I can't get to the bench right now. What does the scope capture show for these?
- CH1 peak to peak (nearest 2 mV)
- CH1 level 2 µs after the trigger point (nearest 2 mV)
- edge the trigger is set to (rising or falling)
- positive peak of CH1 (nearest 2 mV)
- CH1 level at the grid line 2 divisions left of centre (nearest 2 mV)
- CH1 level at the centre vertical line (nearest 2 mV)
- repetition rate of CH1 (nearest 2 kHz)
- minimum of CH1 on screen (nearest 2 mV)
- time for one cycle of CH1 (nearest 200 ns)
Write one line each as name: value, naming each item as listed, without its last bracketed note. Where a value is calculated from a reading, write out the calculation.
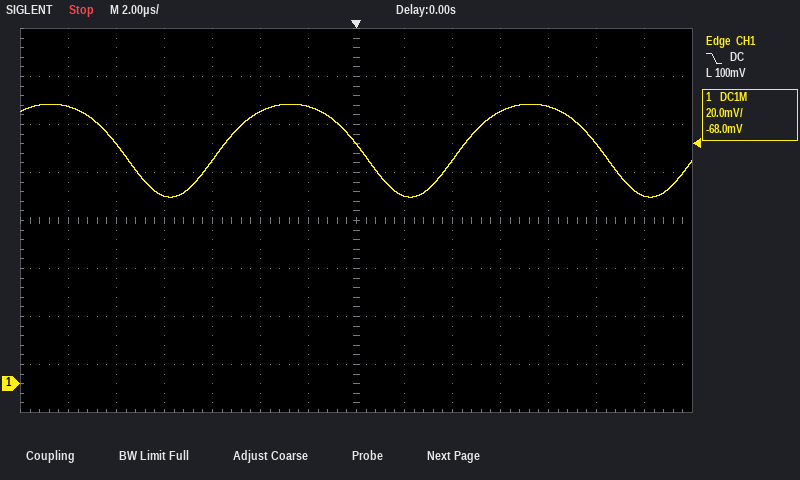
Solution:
CH1 peak to peak: 116 mV − (78 mV) = 38 mV
CH1 level 2 µs after the trigger point: 78 mV
edge the trigger is set to: falling
positive peak of CH1: 116 mV
CH1 level at the grid line 2 divisions left of centre: 114 mV
CH1 level at the centre vertical line: 100 mV
repetition rate of CH1: 1 / 10.0 µs ≈ 100 kHz
minimum of CH1 on screen: 78 mV
time for one cycle of CH1: 10.0 µs
